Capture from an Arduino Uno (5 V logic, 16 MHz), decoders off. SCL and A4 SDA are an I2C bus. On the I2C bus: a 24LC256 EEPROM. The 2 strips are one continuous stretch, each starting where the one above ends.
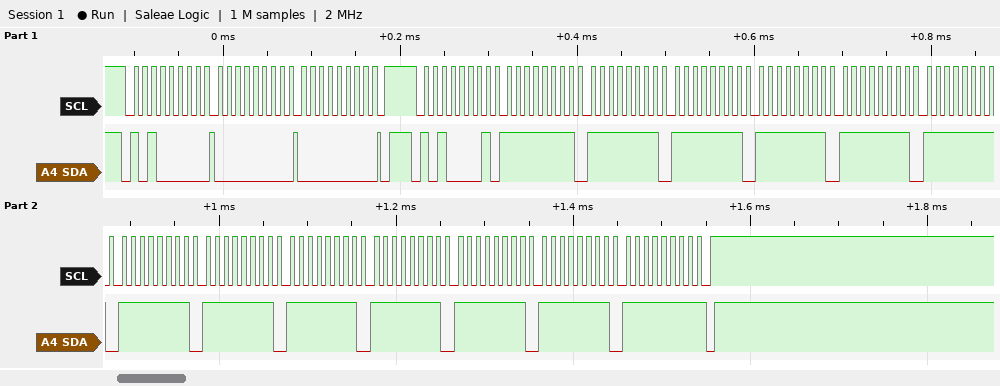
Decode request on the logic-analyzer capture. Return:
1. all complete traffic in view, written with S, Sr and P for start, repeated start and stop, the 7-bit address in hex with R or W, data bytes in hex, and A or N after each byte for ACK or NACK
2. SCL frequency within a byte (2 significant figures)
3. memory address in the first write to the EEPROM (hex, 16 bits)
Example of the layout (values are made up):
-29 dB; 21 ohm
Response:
S 50W A 00 A 00 A P S 50R A FF A FF A FF A FF A FF A FF A FF A FF A FF A FF A FF A FF A FF N P; 100 kHz; 0x0000
